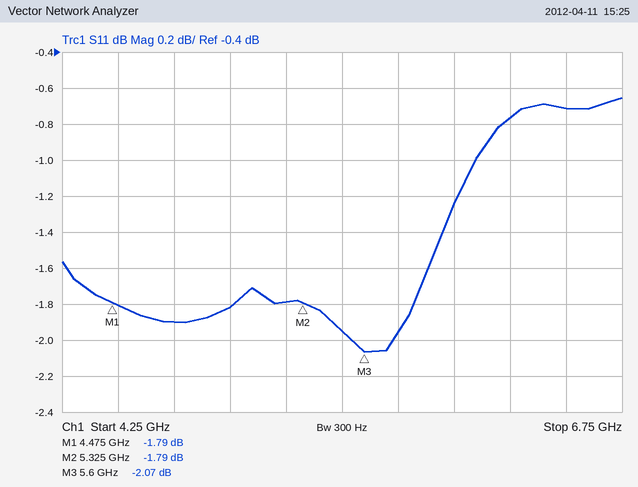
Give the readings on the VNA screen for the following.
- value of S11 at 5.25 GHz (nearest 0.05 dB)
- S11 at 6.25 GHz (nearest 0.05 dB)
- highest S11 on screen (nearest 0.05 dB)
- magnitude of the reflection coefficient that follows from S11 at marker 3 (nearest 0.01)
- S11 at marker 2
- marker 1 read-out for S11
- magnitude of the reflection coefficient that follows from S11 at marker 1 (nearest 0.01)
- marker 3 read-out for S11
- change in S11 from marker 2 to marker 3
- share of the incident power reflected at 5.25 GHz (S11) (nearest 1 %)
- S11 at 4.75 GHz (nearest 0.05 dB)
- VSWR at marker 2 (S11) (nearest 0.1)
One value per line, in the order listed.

-1.80 dB
-0.75 dB
-0.65 dB
0.79
-1.79 dB
-1.79 dB
0.81
-2.07 dB
-0.28 dB
66 %
-1.90 dB
9.7
